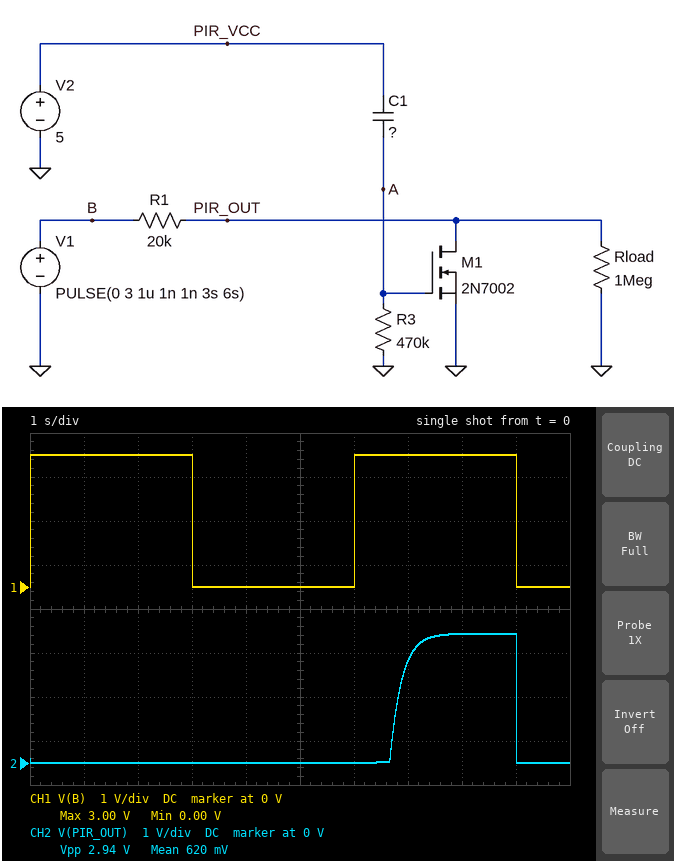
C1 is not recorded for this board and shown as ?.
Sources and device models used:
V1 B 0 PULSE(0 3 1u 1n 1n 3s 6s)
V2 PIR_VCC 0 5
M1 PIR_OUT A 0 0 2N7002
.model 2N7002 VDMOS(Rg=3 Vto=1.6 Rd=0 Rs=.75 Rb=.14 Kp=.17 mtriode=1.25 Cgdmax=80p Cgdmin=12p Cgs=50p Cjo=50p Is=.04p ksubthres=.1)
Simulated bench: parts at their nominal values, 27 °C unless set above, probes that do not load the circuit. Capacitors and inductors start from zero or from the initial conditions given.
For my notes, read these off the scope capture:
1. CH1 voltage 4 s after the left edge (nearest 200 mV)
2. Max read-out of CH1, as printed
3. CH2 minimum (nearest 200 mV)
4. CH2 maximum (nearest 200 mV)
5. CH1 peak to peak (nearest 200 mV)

0 V
3.00 V
0 V
3.0 V
3.0 V
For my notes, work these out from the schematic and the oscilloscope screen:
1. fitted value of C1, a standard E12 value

12 µF
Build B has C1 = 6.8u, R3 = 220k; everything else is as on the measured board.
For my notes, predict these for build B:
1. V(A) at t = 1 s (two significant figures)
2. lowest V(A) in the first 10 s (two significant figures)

2.6 V
6.2 mV
